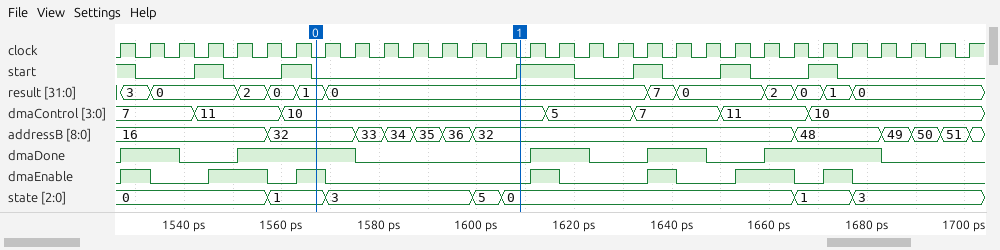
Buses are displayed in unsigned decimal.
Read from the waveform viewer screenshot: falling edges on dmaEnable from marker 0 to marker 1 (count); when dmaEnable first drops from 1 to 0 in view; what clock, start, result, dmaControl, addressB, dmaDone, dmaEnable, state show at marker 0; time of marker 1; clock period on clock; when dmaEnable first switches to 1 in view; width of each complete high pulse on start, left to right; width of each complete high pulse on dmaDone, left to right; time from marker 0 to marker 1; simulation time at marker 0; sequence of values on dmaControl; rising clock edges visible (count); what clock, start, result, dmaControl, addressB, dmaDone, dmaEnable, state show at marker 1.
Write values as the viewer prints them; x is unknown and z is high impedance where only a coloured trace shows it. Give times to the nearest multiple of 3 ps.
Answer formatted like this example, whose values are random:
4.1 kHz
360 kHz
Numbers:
1
1533 ps
clock=0, start=0, result=1, dmaControl=10, addressB=32, dmaDone=1, dmaEnable=1, state=1
1608 ps
6 ps
1527 ps
6 ps, 6 ps, 12 ps, 6 ps, 6 ps, 6 ps
12 ps, 24 ps, 12 ps, 12 ps, 24 ps
42 ps
1566 ps
7, 11, 10, 5, 7, 11, 10
30
clock=0, start=1, result=0, dmaControl=10, addressB=32, dmaDone=0, dmaEnable=0, state=0
